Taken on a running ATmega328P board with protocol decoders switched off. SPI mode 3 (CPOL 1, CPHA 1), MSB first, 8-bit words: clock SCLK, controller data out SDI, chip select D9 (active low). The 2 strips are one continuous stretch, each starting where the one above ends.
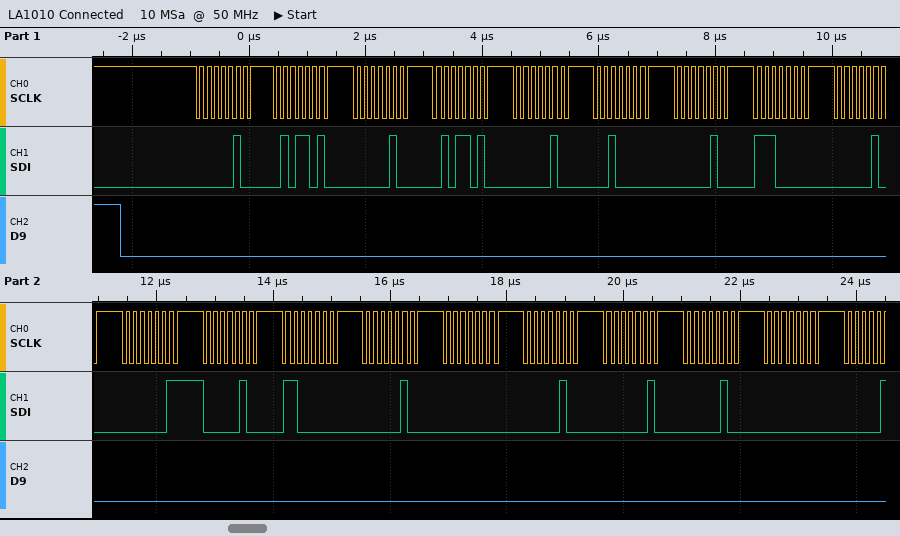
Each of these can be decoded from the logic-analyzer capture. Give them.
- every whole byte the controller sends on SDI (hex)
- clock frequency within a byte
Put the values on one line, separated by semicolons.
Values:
04 5A 04 5A 04 20 04 E0 04 03 04 C0 04 00 04 02 04 00; 8 MHz
